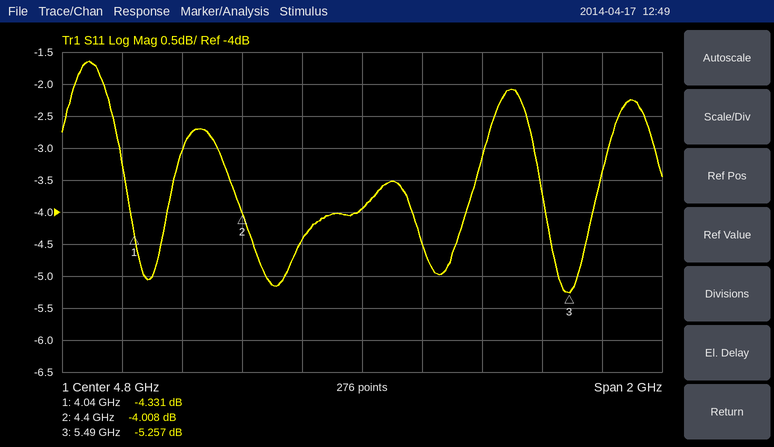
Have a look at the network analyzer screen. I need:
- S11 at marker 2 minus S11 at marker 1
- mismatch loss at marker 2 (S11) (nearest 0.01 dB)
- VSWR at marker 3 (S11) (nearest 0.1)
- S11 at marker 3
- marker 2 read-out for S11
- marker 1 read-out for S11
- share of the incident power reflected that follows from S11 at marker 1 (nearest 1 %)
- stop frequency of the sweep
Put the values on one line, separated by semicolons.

0.323 dB; 2.20 dB; 3.4; -5.257 dB; -4.008 dB; -4.331 dB; 37 %; 5.8 GHz
